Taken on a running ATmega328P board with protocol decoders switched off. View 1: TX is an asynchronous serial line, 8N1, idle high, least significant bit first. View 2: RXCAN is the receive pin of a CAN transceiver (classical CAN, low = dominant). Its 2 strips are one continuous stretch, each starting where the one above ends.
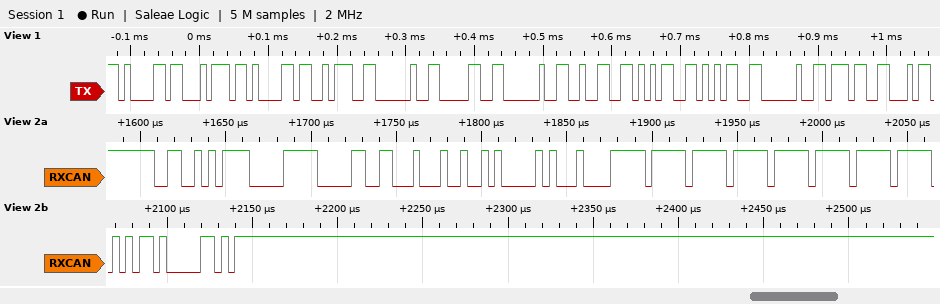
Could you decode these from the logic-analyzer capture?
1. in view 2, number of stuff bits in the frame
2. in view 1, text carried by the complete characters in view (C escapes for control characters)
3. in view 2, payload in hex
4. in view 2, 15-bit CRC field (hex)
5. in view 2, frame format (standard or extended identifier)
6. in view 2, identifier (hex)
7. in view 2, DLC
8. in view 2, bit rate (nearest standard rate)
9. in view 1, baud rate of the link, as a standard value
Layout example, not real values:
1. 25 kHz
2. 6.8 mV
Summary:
1. 13
2. "ata: 0 255 7"
3. 92 81 10 FF FF FF FF FF
4. 0x5682
5. extended
6. 0x0CAC1E13
7. 8
8. 250 kbit/s
9. 115200 baud
